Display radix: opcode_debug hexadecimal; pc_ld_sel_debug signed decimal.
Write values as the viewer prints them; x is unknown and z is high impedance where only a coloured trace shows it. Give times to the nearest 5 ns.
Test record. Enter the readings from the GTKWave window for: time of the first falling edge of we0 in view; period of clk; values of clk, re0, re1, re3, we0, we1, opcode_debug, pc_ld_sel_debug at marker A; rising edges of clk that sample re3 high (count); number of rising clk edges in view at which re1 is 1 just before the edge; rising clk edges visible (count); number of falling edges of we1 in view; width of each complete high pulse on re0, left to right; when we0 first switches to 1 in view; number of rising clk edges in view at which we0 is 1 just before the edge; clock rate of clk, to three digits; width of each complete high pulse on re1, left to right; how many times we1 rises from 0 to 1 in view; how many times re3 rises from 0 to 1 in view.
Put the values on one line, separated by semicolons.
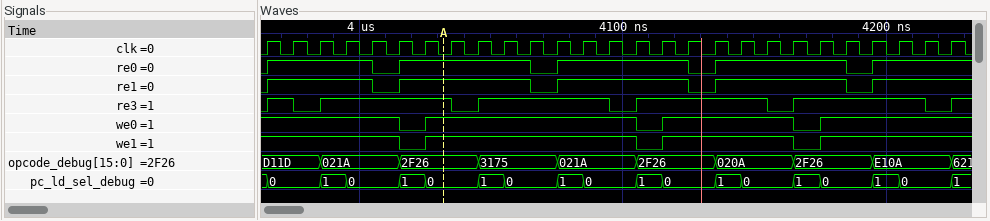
4015 ns; 10 ns; clk=0, re0=1, re1=1, re3=1, we0=1, we1=1, opcode_debug=2F26, pc_ld_sel_debug=0; 21; 22; 27; 3; 40 ns, 50 ns, 50 ns, 50 ns; 4025 ns; 24; 100 MHz; 40 ns, 50 ns, 50 ns, 50 ns; 3; 6
